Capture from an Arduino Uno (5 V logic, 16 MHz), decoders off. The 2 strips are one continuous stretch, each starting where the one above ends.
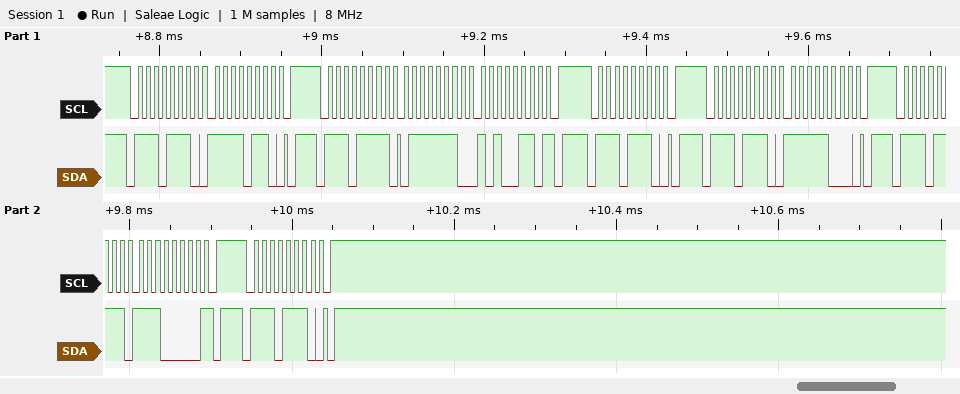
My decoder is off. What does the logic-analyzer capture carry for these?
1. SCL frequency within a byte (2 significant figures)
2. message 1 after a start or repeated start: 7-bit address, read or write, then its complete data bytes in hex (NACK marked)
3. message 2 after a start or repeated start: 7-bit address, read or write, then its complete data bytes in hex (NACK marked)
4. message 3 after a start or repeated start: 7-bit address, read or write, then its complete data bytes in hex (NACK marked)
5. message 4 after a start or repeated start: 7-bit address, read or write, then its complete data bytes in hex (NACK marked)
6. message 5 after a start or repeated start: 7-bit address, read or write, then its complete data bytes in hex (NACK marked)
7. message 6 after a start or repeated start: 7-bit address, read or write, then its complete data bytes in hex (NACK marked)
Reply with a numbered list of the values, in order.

1. 100 kHz
2. 0x77 write: F6
3. 0x77 read: 7E A6 NACK
4. 0x77 write
5. 0x77 write: F8
6. 0x77 read: E0 NACK
7. 0x77 write
